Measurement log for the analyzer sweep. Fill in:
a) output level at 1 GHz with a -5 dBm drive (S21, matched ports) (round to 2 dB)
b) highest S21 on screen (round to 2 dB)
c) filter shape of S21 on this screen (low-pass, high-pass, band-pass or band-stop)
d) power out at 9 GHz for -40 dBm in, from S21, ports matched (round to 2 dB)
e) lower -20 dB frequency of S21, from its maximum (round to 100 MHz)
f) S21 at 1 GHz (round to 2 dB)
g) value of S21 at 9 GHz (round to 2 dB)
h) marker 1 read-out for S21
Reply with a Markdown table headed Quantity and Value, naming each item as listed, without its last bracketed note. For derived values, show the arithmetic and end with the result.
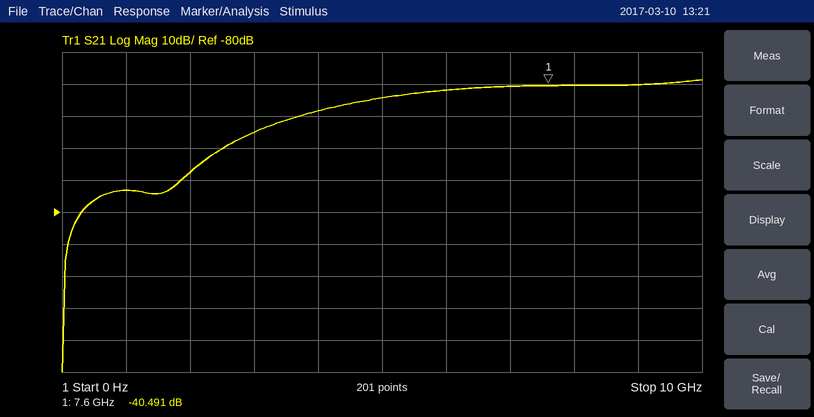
| Quantity | Value |
|---|---|
| output level at 1 GHz with a -5 dBm drive (S21, matched ports) | -5 dBm + (-74 dB) = -78 dBm |
| highest S21 on screen | -38 dB |
| filter shape of S21 on this screen | high-pass |
| power out at 9 GHz for -40 dBm in, from S21, ports matched | -40 dBm + (-40 dB) = -80 dBm |
| lower -20 dB frequency of S21, from its maximum | 2.6 GHz |
| S21 at 1 GHz | -74 dB |
| value of S21 at 9 GHz | -40 dB |
| marker 1 read-out for S21 | -40.491 dB |
